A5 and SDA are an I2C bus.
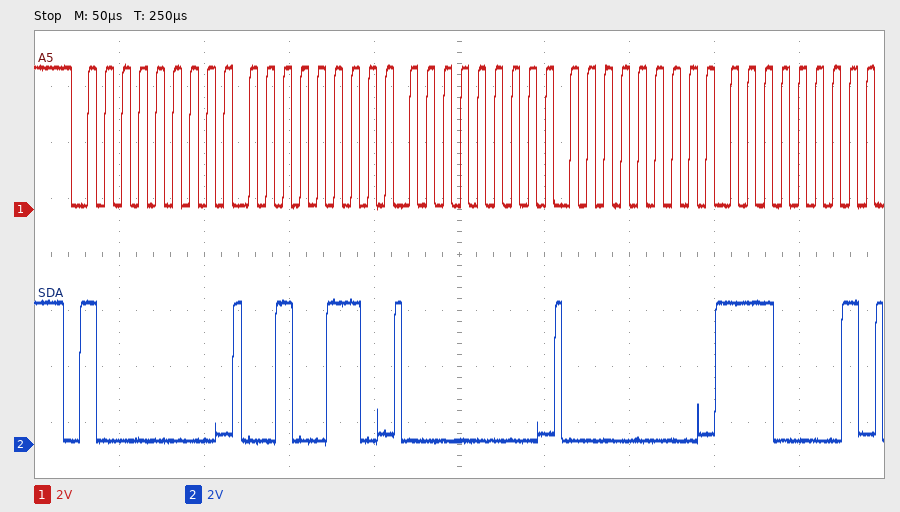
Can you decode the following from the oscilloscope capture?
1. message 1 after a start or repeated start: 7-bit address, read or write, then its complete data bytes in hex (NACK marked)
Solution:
0x40 write: 26 00 00 E1
